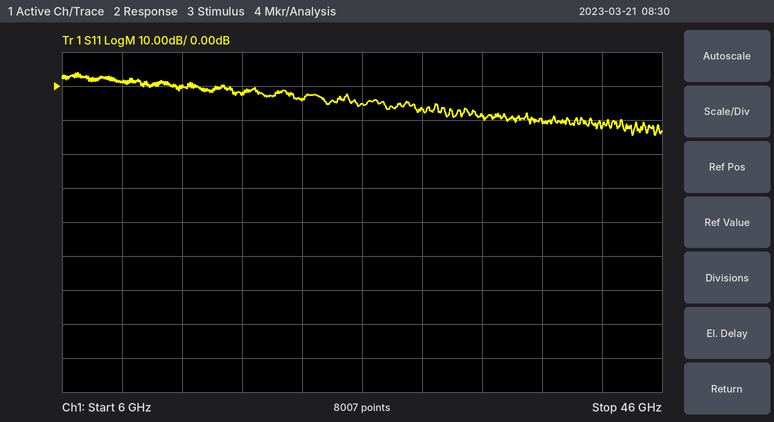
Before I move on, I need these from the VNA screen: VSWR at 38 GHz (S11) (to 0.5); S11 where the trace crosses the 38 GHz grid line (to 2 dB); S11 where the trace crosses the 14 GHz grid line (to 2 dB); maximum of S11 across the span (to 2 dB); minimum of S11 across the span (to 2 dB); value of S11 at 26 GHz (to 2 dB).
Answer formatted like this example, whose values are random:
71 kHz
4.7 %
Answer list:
2.0
-10 dB
0 dB
4 dB
-14 dB
-6 dB
